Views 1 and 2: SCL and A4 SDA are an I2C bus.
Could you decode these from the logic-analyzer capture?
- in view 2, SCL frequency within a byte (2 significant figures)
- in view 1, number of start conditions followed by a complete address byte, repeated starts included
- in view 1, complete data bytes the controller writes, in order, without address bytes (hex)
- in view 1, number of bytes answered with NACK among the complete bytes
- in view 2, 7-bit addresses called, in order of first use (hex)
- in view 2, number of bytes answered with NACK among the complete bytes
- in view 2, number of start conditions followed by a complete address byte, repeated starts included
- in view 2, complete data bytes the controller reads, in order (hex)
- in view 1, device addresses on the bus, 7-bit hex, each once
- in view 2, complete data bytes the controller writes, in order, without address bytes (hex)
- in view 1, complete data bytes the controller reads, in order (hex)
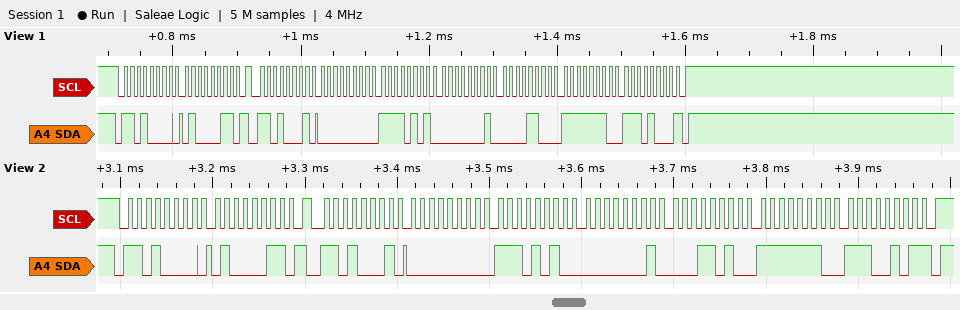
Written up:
100 kHz
2
43
1
0x68
1
2
00 EA 01 1A FE E5
0x68
43
00 F5 01 0C FE E8
